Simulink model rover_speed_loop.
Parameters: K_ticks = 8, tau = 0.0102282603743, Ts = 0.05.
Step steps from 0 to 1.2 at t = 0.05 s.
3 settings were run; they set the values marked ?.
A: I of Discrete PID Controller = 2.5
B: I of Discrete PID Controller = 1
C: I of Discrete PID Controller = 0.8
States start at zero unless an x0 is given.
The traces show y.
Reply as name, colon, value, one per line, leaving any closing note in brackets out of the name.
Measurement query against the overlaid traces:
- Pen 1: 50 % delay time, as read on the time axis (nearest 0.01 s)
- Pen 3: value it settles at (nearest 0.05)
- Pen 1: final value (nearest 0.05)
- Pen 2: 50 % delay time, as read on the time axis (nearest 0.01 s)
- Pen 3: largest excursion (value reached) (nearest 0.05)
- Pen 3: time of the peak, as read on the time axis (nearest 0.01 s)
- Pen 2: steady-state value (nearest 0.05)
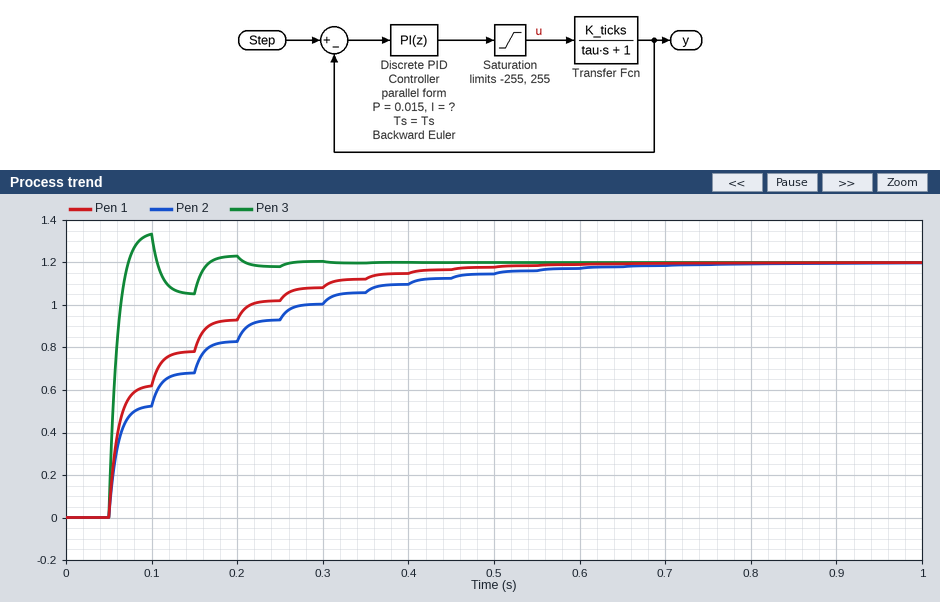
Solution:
Pen 1: 50 % delay time, as read on the time axis: 0.08 s
Pen 3: value it settles at: 1.20
Pen 1: final value: 1.20
Pen 2: 50 % delay time, as read on the time axis: 0.11 s
Pen 3: largest excursion (value reached): 1.35
Pen 3: time of the peak, as read on the time axis: 0.10 s
Pen 2: steady-state value: 1.20
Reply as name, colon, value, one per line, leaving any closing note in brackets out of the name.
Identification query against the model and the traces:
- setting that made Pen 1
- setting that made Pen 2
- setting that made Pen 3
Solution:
setting that made Pen 1: B
setting that made Pen 2: C
setting that made Pen 3: A
